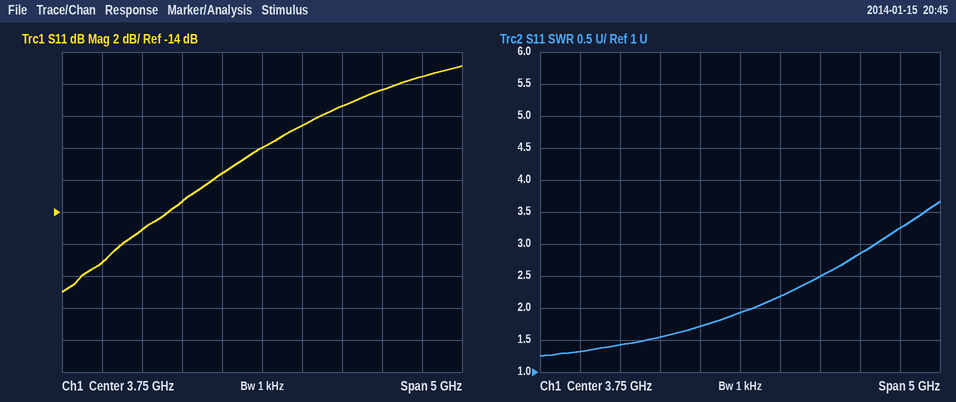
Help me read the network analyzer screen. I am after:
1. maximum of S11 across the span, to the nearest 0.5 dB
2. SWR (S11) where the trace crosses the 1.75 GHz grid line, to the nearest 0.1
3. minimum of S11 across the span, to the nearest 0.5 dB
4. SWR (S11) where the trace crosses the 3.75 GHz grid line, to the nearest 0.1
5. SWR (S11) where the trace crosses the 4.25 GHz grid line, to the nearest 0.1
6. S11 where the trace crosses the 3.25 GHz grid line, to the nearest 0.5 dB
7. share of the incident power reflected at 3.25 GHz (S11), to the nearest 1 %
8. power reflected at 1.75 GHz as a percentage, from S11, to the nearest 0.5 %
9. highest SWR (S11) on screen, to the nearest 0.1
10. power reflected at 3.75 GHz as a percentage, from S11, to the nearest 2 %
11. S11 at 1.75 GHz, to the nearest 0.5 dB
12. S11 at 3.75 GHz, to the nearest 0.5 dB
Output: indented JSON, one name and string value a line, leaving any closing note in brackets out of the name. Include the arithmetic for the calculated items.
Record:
{
  "maximum of S11 across the span, to the nearest 0.5 dB": "-5.0 dB",
  "SWR (S11) where the trace crosses the 1.75 GHz grid line, to the nearest 0.1": "1.3",
  "minimum of S11 across the span, to the nearest 0.5 dB": "-19.0 dB",
  "SWR (S11) where the trace crosses the 3.75 GHz grid line, to the nearest 0.1": "1.9",
  "SWR (S11) where the trace crosses the 4.25 GHz grid line, to the nearest 0.1": "2.2",
  "S11 where the trace crosses the 3.25 GHz grid line, to the nearest 0.5 dB": "-11.5 dB",
  "share of the incident power reflected at 3.25 GHz (S11), to the nearest 1 %": "10^(-11.5/10) ≈ 7 %",
  "power reflected at 1.75 GHz as a percentage, from S11, to the nearest 0.5 %": "10^(-17/10) ≈ 2.0 %",
  "highest SWR (S11) on screen, to the nearest 0.1": "3.7",
  "power reflected at 3.75 GHz as a percentage, from S11, to the nearest 2 %": "10^(-10/10) ≈ 10 %",
  "S11 at 1.75 GHz, to the nearest 0.5 dB": "-17.0 dB",
  "S11 at 3.75 GHz, to the nearest 0.5 dB": "-10.0 dB"
}
